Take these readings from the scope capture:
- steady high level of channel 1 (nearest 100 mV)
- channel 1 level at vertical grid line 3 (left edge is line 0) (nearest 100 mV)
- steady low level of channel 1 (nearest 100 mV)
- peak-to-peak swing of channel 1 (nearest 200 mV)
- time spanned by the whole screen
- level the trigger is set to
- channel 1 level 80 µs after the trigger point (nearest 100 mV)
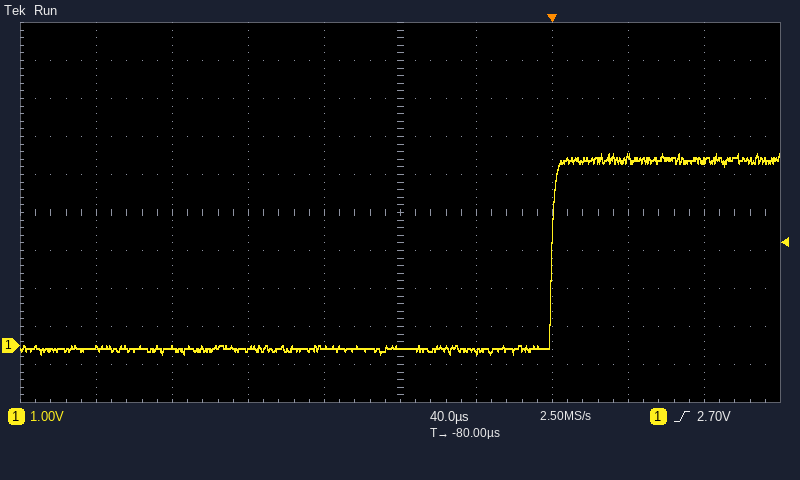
4.9 V
-100 mV
-100 mV
5.2 V
400 µs
2.70 V
4.9 V
